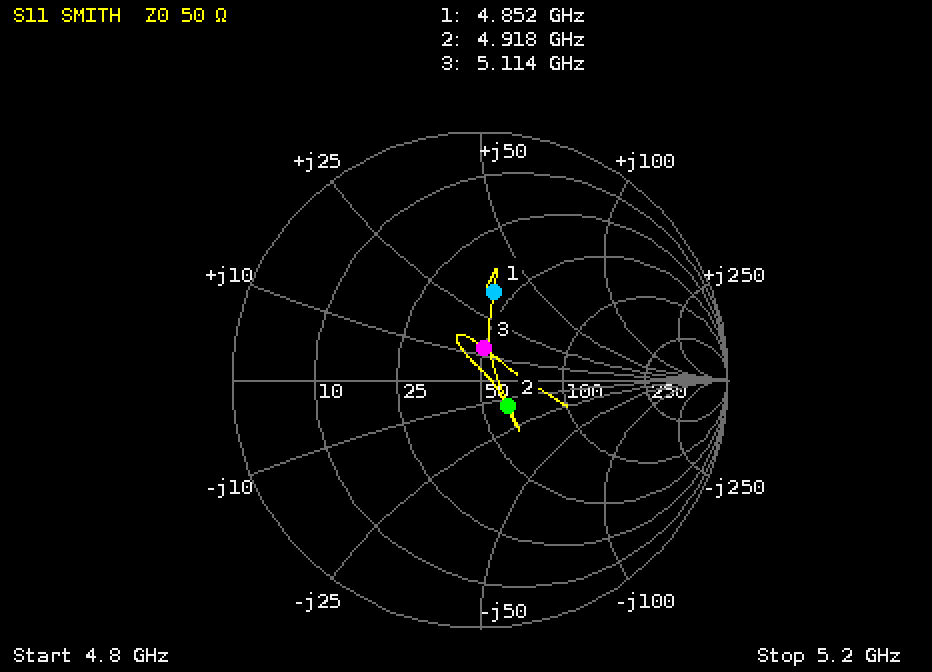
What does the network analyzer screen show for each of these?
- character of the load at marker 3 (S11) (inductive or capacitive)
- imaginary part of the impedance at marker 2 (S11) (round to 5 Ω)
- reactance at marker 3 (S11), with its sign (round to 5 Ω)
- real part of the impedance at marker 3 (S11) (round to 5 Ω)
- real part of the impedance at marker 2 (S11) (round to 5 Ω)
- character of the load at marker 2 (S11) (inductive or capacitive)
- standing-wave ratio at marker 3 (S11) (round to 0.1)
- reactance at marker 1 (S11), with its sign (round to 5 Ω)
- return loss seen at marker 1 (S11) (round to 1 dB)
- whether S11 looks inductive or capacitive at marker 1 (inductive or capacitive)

inductive
-15 Ω
+15 Ω
50 Ω
60 Ω
capacitive
1.3
+35 Ω
9 dB
inductive
